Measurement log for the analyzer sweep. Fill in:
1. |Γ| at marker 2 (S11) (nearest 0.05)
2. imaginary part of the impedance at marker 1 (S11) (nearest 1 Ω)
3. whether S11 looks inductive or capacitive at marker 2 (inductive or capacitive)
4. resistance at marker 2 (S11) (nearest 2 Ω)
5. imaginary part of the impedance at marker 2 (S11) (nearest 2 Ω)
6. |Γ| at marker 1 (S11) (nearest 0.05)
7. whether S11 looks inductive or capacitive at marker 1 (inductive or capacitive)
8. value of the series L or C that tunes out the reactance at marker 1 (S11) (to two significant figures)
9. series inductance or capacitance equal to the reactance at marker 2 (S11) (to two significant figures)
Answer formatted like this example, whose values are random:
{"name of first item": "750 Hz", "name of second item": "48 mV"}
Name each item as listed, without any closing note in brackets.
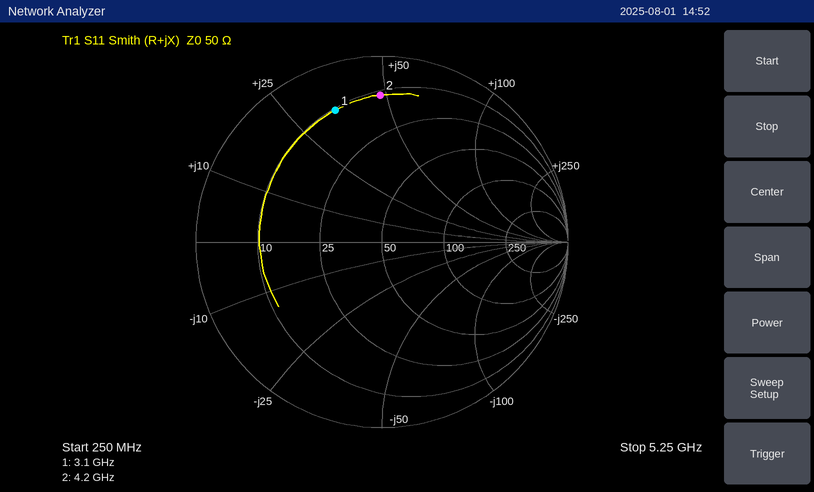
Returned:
{"|Γ| at marker 2 (S11)": "0.80", "imaginary part of the impedance at marker 1 (S11)": "+34 Ω", "whether S11 looks inductive or capacitive at marker 2": "inductive", "resistance at marker 2 (S11)": "12 Ω", "imaginary part of the impedance at marker 2 (S11)": "+48 Ω", "|Γ| at marker 1 (S11)": "0.75", "whether S11 looks inductive or capacitive at marker 1": "inductive", "value of the series L or C that tunes out the reactance at marker 1 (S11)": "1.5 pF", "series inductance or capacitance equal to the reactance at marker 2 (S11)": "1.8 nH"}
